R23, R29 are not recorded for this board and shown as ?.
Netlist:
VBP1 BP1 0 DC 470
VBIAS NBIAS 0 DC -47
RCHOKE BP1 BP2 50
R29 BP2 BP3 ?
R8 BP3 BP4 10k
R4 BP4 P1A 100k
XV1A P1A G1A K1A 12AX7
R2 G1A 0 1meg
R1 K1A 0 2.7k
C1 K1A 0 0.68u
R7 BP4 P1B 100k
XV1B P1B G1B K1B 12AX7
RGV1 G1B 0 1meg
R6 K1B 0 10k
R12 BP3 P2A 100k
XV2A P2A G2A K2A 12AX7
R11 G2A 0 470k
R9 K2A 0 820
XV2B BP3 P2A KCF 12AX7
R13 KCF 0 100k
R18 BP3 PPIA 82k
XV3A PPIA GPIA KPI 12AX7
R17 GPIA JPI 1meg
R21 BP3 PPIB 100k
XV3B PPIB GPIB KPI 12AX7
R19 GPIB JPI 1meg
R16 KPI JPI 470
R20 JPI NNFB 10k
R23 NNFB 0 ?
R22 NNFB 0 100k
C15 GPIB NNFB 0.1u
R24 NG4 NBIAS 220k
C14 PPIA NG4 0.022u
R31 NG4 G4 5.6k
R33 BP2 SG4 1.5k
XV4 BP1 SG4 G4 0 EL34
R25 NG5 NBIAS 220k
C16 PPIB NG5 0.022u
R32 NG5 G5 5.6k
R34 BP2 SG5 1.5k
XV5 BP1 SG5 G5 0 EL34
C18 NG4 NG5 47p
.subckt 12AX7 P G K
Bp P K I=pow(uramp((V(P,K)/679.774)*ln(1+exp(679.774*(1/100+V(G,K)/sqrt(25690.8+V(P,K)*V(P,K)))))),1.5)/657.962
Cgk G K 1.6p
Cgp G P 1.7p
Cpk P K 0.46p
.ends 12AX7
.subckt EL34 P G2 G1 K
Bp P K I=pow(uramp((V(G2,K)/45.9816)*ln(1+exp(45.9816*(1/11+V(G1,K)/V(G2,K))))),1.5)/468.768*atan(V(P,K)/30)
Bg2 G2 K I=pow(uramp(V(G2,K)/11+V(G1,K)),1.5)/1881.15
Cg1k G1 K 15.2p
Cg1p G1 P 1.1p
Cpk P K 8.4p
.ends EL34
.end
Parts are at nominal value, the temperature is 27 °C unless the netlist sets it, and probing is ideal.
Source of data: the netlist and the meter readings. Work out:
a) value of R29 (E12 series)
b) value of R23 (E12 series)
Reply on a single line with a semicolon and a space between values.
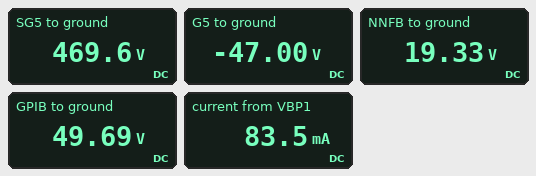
8.2 kΩ; 6.8 kΩ
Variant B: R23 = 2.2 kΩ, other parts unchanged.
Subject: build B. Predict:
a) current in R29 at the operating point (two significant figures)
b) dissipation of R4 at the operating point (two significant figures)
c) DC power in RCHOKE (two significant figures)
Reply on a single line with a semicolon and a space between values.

8.5 mA; 90 mW; 3.6 mW
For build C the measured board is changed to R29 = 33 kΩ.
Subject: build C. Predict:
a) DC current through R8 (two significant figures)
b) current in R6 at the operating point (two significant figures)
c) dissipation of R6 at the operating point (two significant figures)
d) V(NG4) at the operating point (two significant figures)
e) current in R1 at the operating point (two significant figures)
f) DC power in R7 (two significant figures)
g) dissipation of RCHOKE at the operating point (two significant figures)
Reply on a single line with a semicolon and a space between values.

950 µA; 270 µA; 730 µW; -47 V; 680 µA; 7.3 mW; 1.7 mW
